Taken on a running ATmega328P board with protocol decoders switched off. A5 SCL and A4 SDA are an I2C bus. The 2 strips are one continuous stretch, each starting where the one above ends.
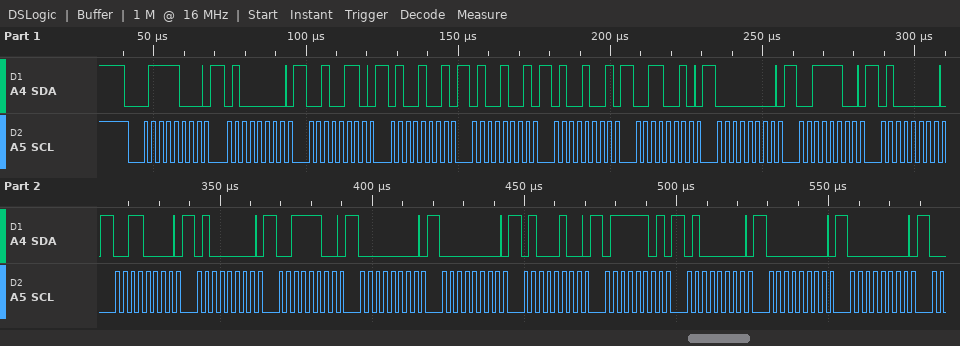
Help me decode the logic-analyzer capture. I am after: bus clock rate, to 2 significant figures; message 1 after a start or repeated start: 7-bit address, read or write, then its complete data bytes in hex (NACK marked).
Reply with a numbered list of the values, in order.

1. 400 kHz
2. 0x3C write: 40 26 49 49 49 32 00 3C 40 30 40 3C 00 00 44 7D 40 00 00
